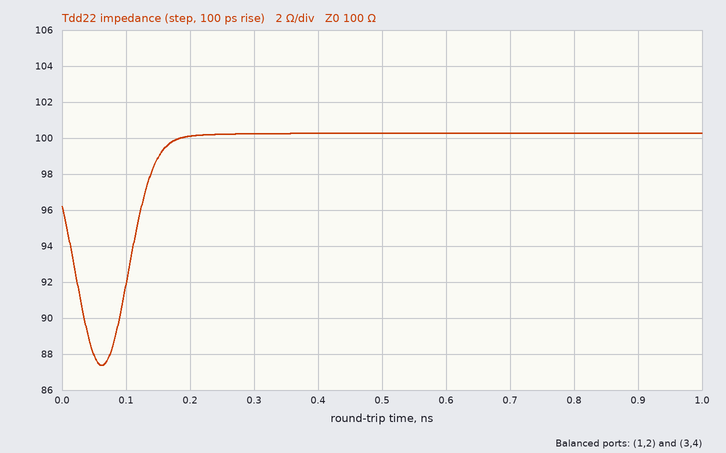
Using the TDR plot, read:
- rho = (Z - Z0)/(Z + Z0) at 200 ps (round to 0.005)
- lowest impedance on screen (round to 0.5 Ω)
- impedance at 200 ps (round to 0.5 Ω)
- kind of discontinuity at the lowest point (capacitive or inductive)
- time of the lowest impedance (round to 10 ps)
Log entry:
0.000
87.5 Ω
100.0 Ω
capacitive
60 ps
